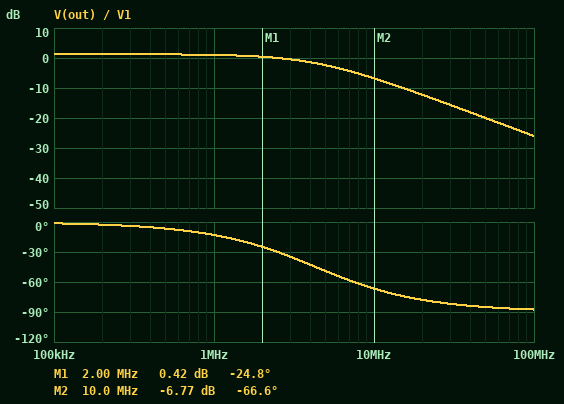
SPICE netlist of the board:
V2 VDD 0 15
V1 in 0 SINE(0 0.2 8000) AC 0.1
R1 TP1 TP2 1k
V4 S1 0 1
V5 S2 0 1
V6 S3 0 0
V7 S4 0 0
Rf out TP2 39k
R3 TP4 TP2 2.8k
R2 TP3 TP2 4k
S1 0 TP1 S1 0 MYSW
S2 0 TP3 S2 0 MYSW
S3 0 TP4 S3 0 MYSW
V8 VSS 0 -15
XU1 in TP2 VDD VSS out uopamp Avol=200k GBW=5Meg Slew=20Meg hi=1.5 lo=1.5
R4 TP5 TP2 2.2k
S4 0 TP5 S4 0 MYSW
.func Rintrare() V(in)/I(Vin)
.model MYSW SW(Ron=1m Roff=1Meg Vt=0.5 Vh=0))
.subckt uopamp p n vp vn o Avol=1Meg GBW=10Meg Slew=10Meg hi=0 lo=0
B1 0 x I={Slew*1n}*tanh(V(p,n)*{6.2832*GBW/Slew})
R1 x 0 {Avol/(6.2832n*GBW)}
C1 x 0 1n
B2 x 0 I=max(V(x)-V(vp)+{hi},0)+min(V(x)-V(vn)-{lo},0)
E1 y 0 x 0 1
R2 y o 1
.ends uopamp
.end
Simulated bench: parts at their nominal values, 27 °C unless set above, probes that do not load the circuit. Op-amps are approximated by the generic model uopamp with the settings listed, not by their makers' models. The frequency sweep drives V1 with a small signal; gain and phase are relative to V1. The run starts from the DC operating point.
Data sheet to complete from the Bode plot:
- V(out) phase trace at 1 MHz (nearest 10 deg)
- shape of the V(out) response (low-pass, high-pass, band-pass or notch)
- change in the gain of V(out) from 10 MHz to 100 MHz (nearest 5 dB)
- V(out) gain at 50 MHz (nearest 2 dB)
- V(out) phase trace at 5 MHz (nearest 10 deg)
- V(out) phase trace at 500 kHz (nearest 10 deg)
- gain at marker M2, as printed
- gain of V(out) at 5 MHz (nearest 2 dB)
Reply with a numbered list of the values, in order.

1. -10 deg
2. low-pass
3. -20 dB
4. -20 dB
5. -50 deg
6. -10 deg
7. -6.77 dB
8. -2 dB
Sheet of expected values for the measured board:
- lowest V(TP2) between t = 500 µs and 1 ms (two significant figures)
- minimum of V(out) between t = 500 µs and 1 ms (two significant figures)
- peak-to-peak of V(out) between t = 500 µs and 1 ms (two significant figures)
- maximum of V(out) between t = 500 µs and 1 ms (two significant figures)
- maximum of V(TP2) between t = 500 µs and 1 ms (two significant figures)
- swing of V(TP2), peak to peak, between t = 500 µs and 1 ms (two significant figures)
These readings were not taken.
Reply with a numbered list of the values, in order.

1. -200 mV
2. -9.9 V
3. 20 V
4. 9.9 V
5. 200 mV
6. 400 mV
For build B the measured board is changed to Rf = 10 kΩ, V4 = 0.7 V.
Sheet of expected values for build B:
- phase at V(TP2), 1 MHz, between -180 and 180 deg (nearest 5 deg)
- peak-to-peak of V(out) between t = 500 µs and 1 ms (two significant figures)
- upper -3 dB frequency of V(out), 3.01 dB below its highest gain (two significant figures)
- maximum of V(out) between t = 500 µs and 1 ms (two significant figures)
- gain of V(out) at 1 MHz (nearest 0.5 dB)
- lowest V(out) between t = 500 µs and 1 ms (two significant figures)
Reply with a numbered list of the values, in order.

1. -10 deg
2. 5.4 V
3. 4.8 MHz
4. 2.7 V
5. 0 dB
6. -2.7 V
